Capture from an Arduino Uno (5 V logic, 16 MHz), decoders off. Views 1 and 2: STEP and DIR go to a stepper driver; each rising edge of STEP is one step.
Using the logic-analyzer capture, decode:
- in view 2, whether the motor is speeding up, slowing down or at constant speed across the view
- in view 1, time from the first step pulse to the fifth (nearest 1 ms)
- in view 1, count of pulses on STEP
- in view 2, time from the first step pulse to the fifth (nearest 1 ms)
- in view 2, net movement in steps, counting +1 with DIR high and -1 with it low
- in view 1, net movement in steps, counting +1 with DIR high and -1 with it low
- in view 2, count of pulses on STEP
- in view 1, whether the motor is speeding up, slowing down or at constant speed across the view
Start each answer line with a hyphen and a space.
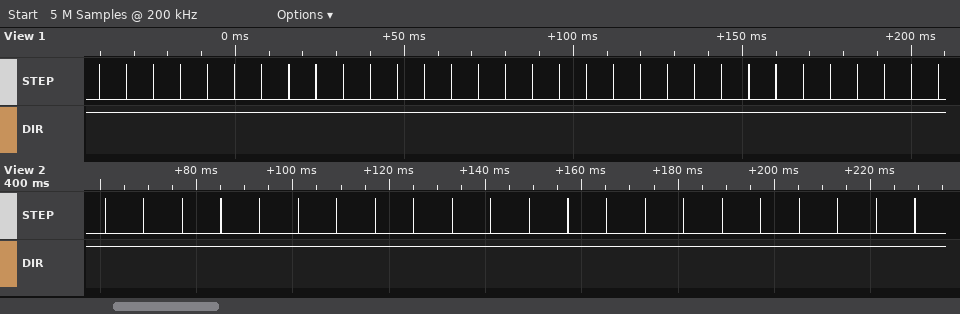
- constant speed
- 32 ms
- 32
- 32 ms
- +22
- +32
- 22
- constant speed
